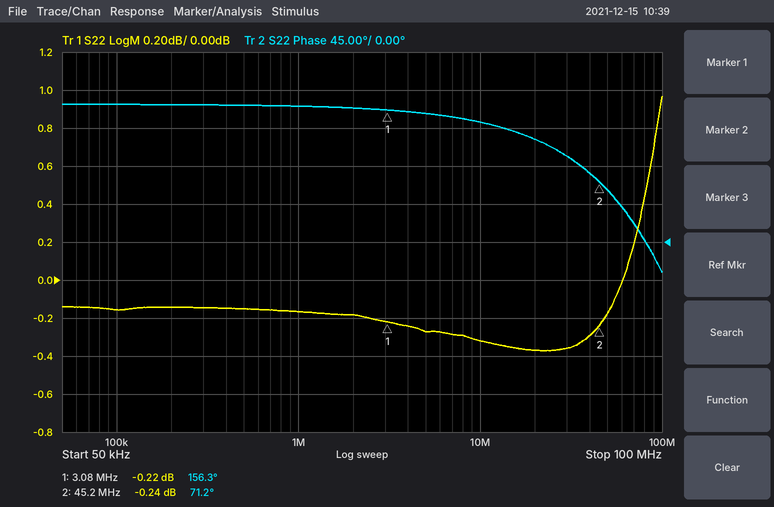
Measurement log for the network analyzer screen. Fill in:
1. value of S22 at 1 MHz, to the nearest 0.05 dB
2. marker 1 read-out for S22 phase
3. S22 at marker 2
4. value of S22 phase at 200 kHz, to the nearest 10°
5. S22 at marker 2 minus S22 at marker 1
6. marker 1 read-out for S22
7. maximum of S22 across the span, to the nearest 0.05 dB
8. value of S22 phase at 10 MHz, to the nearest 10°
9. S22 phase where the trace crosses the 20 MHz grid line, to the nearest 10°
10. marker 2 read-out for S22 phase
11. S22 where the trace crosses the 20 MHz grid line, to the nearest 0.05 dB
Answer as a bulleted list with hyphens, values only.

- -0.15 dB
- 156.3°
- -0.24 dB
- 160°
- -0.02 dB
- -0.22 dB
- 0.95 dB
- 140°
- 120°
- 71.2°
- -0.35 dB
